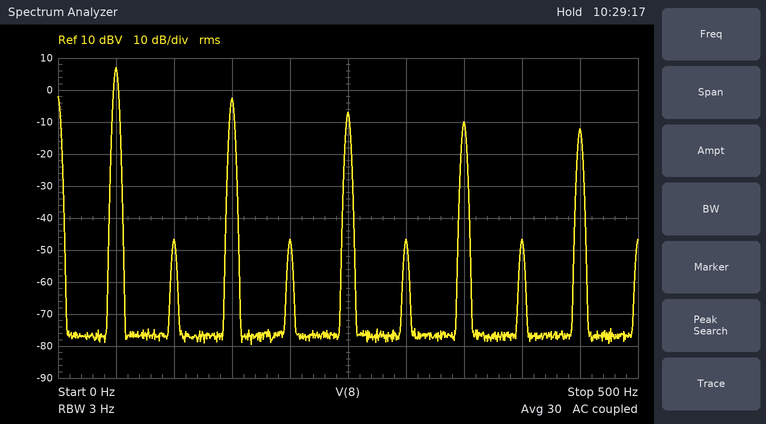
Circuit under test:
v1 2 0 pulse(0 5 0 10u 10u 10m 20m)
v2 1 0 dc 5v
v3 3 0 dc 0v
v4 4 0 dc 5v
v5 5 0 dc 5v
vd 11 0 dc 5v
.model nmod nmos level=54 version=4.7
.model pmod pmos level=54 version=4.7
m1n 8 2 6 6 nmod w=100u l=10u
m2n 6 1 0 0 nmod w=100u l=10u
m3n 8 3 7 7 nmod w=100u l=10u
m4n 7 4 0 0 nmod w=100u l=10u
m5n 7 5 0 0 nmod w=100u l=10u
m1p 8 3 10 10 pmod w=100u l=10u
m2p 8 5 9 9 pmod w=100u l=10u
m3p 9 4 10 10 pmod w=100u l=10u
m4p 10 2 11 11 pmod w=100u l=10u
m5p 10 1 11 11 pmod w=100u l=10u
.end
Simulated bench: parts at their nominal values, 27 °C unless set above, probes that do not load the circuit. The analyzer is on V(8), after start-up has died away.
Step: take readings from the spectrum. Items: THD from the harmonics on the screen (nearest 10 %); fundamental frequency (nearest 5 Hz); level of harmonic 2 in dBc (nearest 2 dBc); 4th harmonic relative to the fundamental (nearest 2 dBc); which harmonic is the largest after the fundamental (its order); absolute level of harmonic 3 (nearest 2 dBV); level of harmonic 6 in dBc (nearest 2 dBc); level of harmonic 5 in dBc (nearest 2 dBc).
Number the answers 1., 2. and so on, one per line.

1. 40 %
2. 50 Hz
3. -54 dBc
4. -54 dBc
5. 3
6. -2 dBV
7. -54 dBc
8. -14 dBc
